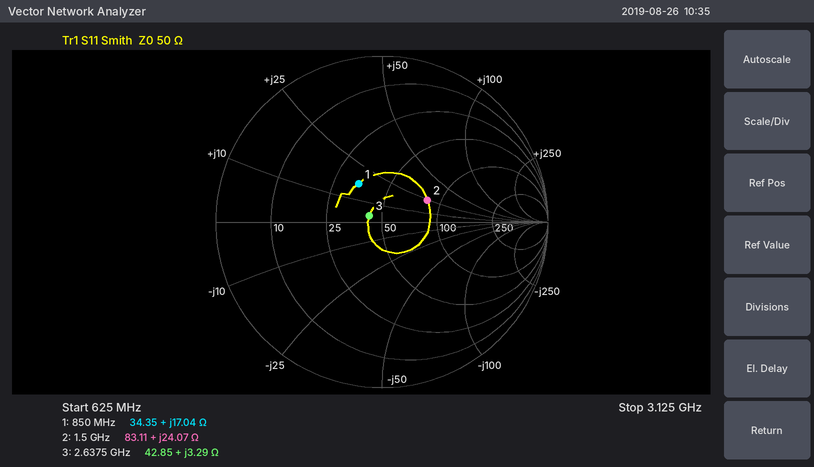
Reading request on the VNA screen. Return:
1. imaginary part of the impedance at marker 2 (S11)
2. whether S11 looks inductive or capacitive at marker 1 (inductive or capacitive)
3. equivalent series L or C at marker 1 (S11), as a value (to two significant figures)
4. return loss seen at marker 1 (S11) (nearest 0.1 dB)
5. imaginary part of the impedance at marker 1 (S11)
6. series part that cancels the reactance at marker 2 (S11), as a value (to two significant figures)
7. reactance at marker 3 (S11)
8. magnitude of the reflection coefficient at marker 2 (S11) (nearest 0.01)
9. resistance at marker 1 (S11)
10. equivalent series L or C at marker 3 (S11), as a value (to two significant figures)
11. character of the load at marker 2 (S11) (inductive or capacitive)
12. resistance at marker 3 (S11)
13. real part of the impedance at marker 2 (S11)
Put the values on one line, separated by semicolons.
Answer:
+24.07 Ω; inductive; 3.2 nH; 11.4 dB; +17.04 Ω; 4.4 pF; +3.29 Ω; 0.30; 34.35 Ω; 200 pH; inductive; 42.85 Ω; 83.11 Ω
